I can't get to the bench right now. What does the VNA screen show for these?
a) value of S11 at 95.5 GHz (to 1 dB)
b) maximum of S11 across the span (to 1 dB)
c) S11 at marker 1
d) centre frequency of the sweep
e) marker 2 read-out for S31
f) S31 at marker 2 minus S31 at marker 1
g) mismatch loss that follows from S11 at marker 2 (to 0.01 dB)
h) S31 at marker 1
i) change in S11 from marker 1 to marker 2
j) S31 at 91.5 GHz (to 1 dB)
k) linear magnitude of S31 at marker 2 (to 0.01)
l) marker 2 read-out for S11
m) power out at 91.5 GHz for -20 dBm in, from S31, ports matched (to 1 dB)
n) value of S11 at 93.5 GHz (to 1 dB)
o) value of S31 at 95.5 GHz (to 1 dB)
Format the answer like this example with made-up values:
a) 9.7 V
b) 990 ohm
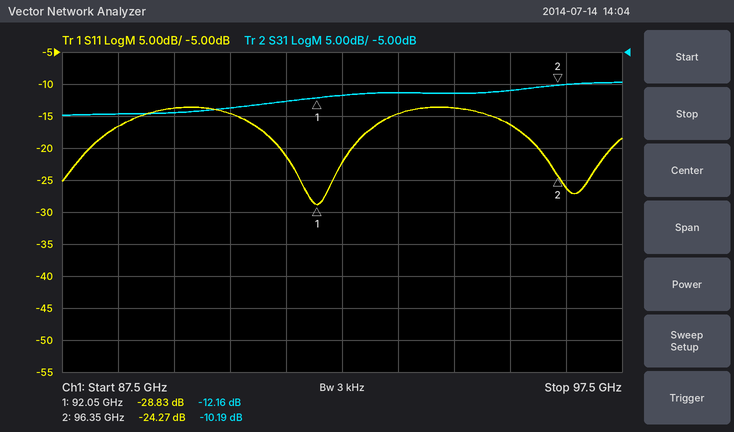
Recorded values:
a) -16 dB
b) -14 dB
c) -28.83 dB
d) 92.5 GHz
e) -10.19 dB
f) 1.97 dB
g) 0.02 dB
h) -12.16 dB
i) 4.56 dB
j) -13 dB
k) 0.31
l) -24.27 dB
m) -33 dBm
n) -15 dB
o) -11 dB
